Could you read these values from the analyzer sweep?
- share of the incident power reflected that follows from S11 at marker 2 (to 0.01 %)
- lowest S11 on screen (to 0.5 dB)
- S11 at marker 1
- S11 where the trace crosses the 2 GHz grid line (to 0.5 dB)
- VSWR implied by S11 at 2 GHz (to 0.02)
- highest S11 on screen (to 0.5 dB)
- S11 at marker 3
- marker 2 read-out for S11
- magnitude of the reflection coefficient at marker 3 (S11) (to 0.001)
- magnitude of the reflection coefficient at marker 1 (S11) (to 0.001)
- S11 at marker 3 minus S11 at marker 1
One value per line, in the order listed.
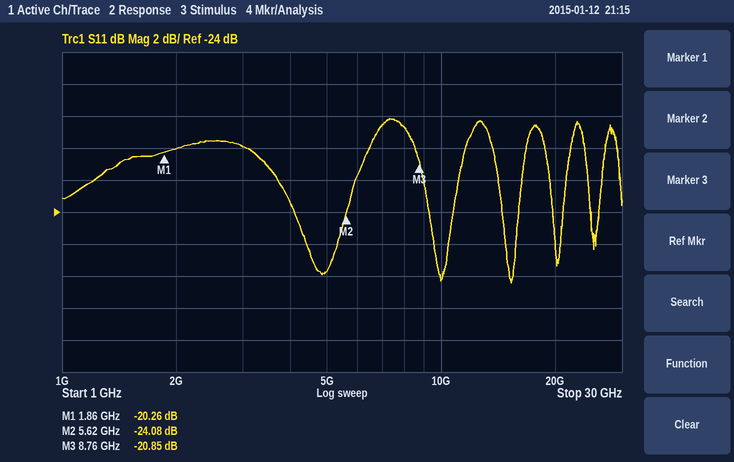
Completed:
0.39 %
-28.5 dB
-20.26 dB
-20.0 dB
1.22
-18.0 dB
-20.85 dB
-24.08 dB
0.091
0.097
-0.59 dB
